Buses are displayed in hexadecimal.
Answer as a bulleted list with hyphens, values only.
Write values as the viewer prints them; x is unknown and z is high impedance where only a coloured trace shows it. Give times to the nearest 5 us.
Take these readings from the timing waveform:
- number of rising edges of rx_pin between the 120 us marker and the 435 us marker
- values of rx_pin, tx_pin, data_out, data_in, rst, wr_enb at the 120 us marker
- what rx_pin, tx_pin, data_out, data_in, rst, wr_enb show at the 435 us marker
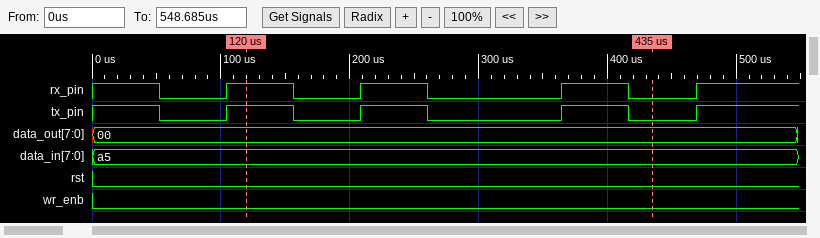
- 2
- rx_pin=1, tx_pin=1, data_out=00, data_in=a5, rst=0, wr_enb=0
- rx_pin=0, tx_pin=0, data_out=00, data_in=a5, rst=0, wr_enb=0
